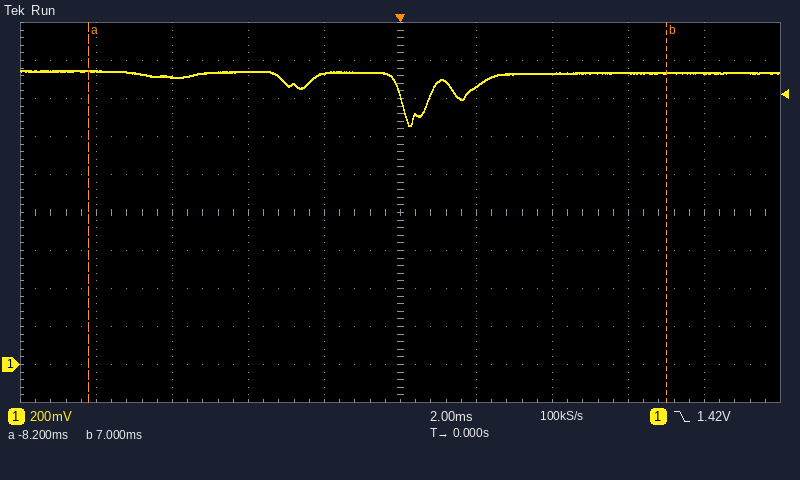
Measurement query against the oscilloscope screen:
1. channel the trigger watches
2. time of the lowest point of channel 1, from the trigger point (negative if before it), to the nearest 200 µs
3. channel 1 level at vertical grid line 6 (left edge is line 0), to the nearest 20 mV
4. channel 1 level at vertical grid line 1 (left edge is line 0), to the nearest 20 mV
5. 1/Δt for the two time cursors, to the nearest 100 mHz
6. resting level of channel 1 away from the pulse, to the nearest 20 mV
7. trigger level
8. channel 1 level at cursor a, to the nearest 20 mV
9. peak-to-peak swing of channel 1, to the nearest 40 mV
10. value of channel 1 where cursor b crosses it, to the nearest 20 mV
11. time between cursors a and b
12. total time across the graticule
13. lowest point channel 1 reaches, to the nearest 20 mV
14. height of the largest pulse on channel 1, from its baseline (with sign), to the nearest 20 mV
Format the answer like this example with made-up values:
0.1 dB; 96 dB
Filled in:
channel 1; +200 µs; 1.46 V; 1.54 V; 65.8 Hz; 1.54 V; 1.42 V; 1.54 V; 280 mV; 1.54 V; 15.2 ms; 20 ms; 1.26 V; -280 mV
